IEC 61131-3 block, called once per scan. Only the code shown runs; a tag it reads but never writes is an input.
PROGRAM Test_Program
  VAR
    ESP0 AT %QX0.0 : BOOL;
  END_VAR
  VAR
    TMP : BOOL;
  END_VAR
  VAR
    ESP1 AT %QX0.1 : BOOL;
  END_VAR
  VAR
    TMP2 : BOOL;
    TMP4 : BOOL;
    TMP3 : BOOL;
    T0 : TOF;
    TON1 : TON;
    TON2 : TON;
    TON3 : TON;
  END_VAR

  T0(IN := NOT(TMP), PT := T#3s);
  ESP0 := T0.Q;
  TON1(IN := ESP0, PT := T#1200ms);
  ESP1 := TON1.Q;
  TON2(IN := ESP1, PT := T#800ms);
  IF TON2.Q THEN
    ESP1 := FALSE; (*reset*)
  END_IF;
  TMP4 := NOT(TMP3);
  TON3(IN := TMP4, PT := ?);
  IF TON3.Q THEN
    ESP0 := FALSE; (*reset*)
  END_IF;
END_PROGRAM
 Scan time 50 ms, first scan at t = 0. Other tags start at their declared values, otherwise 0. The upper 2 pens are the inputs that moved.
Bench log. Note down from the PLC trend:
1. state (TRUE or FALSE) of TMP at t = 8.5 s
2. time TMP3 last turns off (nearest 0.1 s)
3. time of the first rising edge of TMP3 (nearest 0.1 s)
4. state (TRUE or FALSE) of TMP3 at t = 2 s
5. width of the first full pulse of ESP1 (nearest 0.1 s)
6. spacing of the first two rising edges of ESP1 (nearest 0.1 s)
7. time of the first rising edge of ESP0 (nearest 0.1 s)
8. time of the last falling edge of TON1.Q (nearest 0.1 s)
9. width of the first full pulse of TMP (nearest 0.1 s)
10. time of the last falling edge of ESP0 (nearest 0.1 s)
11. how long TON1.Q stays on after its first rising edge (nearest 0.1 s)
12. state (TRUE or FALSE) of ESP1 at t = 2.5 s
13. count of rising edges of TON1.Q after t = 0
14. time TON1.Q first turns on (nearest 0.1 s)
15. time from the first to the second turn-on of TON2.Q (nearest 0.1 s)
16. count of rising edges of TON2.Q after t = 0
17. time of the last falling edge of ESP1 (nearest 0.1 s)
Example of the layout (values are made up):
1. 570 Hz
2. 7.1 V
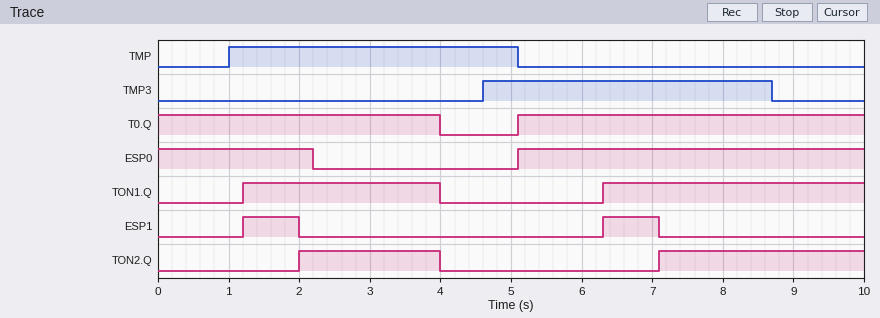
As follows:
1. FALSE
2. 8.7 s
3. 4.6 s
4. FALSE
5. 0.8 s
6. 5.1 s
7. 5.1 s
8. 4.0 s
9. 4.1 s
10. 2.2 s
11. 2.8 s
12. FALSE
13. 2
14. 1.2 s
15. 5.1 s
16. 2
17. 7.1 s
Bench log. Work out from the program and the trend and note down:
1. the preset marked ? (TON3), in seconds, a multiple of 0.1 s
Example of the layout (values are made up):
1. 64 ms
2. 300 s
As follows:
1. 2.2 s
